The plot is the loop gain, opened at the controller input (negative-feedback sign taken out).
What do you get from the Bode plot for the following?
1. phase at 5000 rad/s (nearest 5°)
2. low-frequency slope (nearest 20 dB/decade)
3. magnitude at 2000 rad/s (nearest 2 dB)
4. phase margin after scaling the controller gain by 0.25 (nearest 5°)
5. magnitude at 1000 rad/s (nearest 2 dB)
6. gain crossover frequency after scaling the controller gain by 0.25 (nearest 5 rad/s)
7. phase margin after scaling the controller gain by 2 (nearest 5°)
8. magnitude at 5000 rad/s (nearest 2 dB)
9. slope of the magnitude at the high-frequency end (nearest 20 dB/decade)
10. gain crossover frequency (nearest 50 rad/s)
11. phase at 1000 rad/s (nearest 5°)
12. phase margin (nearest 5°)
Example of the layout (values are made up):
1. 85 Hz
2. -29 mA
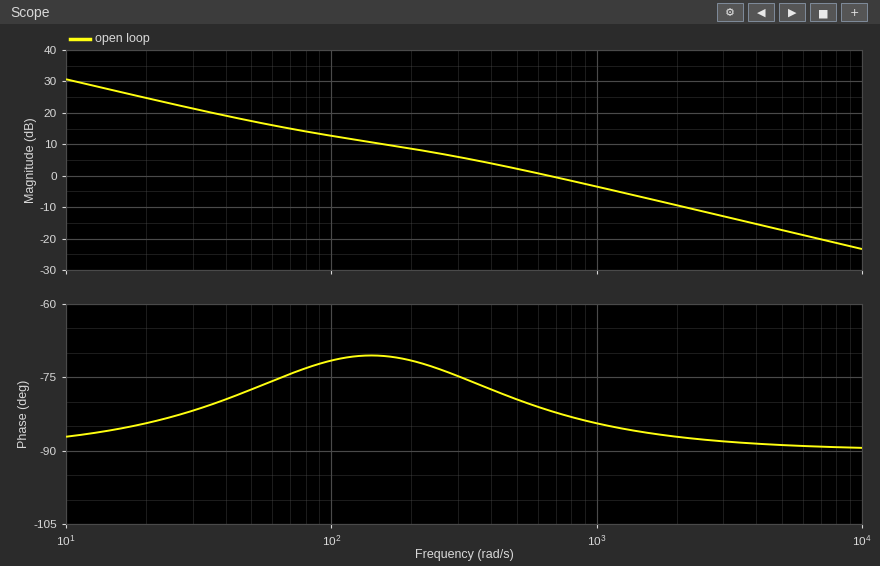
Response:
1. -90°
2. -20 dB/decade
3. -10 dB
4. 110°
5. -4 dB
6. 110 rad/s
7. 95°
8. -18 dB
9. -20 dB/decade
10. 650 rad/s
11. -85°
12. 100°
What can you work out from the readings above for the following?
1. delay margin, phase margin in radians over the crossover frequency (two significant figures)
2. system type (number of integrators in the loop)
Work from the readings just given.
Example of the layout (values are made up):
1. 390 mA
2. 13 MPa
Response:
1. 0.0027 s
2. 1
